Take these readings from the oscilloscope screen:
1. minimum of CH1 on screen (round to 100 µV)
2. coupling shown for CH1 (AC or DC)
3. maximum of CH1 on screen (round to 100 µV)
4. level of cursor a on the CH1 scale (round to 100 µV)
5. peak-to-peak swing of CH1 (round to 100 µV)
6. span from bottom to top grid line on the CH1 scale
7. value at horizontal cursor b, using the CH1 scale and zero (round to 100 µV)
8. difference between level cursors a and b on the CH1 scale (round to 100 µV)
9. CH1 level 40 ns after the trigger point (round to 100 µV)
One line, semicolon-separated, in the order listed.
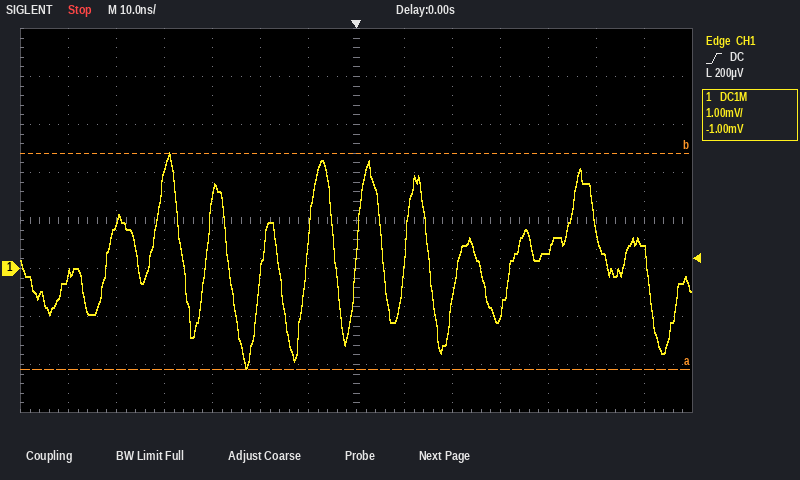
-2.1 mV; DC; 2.4 mV; -2.1 mV; 4.5 mV; 8 mV; 2.4 mV; 4.5 mV; 400 µV
